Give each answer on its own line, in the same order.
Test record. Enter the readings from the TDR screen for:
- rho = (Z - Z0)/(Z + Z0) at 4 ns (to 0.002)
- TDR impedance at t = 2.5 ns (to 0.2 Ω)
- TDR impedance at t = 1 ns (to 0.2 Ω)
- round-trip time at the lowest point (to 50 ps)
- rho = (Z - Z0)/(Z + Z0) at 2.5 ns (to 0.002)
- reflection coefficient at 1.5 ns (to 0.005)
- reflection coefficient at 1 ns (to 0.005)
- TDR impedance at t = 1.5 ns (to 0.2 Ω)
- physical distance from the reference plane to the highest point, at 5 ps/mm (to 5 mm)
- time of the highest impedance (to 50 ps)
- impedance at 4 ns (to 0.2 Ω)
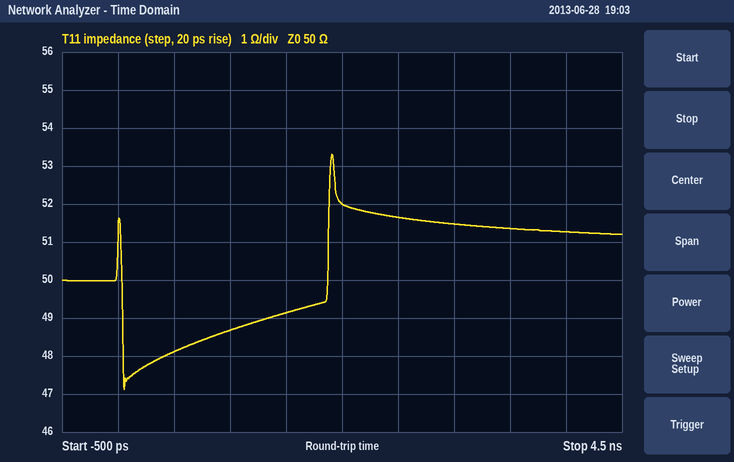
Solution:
+0.012
51.6 Ω
48.6 Ω
50 ps
+0.016
-0.010
-0.015
49.2 Ω
190 mm
1.90 ns
51.2 Ω
